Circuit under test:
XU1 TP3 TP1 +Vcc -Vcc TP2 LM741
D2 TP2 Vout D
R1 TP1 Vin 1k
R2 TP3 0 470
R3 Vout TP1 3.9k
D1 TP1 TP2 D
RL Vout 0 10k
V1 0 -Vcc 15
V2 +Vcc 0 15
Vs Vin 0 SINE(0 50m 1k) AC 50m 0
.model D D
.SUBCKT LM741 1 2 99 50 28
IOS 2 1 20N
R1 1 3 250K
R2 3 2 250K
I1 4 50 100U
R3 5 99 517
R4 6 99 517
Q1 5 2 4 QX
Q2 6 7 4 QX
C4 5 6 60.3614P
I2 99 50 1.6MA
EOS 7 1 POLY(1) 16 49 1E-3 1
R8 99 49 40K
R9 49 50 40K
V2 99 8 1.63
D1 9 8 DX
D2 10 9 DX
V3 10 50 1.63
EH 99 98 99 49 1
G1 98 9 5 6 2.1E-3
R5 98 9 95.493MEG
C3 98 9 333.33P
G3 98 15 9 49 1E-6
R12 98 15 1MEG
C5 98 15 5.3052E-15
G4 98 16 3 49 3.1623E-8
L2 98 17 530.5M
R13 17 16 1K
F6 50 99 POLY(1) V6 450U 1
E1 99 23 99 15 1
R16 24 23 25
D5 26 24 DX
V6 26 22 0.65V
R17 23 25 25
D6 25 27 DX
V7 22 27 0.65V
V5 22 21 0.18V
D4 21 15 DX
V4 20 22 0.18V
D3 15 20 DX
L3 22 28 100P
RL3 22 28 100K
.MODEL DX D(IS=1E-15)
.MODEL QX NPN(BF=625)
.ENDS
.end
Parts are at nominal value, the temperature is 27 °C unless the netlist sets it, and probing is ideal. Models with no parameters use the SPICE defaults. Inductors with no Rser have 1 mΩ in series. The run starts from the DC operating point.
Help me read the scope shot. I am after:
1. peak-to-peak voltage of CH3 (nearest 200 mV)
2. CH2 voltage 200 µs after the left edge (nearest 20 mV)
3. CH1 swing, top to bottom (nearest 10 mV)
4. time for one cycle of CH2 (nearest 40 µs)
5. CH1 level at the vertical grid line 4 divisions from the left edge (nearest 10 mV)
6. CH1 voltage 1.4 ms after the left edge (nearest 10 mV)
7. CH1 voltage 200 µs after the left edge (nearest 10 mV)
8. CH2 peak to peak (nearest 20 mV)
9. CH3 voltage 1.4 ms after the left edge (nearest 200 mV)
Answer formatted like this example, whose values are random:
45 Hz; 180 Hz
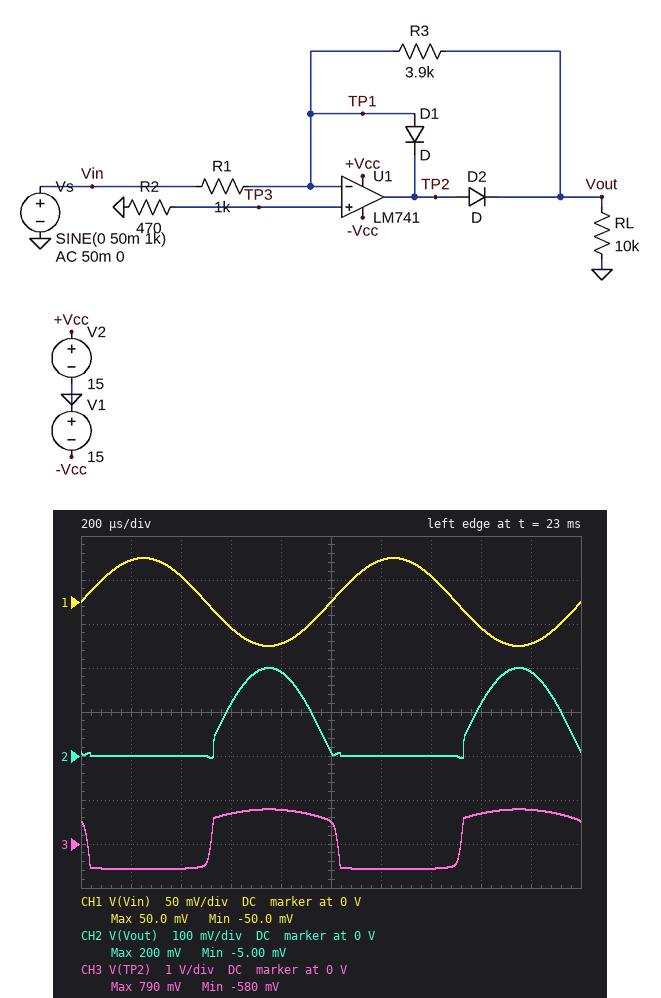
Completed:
1.4 V; 0 V; 100 mV; 1.00 ms; -50 mV; 30 mV; 50 mV; 200 mV; -600 mV
